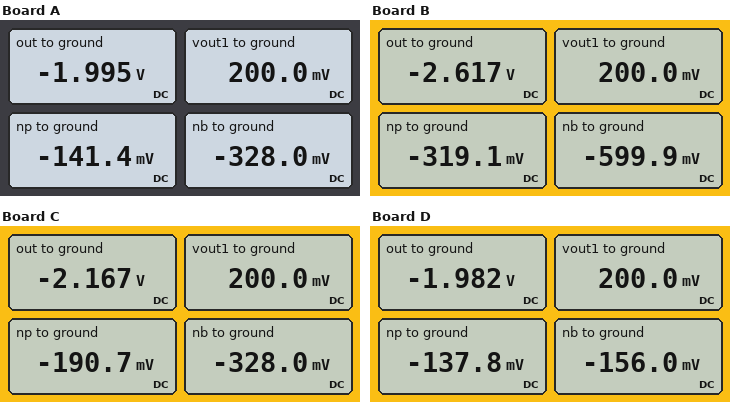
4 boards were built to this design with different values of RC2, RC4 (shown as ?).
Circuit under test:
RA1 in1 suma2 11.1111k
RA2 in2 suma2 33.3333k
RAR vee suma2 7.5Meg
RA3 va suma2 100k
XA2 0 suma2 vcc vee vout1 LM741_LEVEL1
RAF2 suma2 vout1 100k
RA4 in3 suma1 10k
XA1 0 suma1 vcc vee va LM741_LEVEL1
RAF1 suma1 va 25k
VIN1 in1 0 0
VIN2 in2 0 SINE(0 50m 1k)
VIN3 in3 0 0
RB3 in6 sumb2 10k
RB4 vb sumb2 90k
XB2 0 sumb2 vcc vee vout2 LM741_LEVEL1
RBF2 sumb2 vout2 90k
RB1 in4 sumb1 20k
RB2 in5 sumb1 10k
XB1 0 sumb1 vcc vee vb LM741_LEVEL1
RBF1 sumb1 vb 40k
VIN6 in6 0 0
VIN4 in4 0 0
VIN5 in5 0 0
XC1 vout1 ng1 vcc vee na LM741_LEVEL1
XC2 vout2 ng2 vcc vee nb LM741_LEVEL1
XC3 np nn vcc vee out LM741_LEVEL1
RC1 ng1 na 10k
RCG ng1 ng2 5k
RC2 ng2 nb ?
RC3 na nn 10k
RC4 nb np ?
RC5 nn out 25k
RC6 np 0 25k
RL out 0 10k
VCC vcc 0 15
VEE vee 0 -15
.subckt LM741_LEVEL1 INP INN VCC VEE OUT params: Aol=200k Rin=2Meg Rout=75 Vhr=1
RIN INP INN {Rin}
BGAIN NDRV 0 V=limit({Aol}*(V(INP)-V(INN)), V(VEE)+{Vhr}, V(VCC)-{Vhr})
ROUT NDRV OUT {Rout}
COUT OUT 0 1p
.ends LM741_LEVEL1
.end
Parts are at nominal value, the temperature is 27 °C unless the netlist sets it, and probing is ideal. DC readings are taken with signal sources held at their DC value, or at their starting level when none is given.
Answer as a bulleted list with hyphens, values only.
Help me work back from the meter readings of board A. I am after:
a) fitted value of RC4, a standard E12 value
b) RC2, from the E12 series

- 33 kΩ
- 8.2 kΩ
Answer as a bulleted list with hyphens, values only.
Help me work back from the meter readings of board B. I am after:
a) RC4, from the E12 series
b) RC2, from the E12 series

- 22 kΩ
- 15 kΩ
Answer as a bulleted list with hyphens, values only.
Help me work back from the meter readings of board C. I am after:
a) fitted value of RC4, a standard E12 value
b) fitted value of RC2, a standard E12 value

- 18 kΩ
- 8.2 kΩ
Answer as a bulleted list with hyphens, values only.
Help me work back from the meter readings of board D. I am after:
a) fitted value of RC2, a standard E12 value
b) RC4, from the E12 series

- 3.9 kΩ
- 3.3 kΩ
